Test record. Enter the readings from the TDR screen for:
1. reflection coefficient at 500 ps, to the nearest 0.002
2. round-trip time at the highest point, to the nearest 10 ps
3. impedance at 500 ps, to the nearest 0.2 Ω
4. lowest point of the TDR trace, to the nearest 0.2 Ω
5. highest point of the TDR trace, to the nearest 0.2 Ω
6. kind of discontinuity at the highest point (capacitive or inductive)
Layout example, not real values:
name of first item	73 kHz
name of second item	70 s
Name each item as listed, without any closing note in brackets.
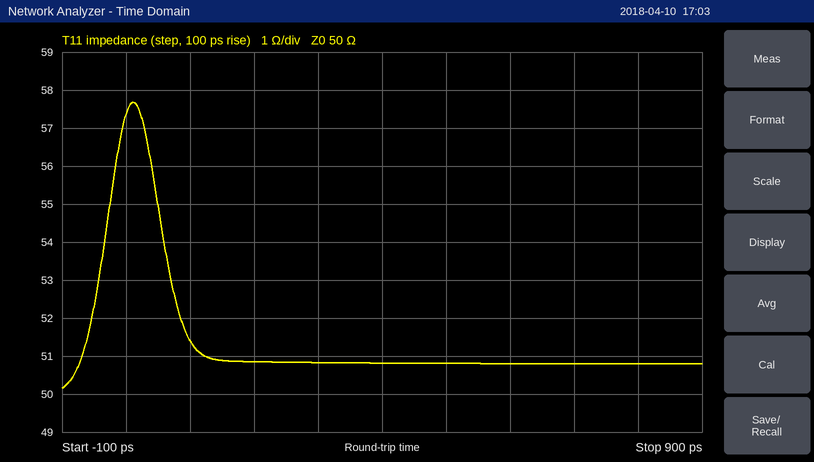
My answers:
reflection coefficient at 500 ps, to the nearest 0.002	+0.008
round-trip time at the highest point, to the nearest 10 ps	10 ps
impedance at 500 ps, to the nearest 0.2 Ω	50.8 Ω
lowest point of the TDR trace, to the nearest 0.2 Ω	50.2 Ω
highest point of the TDR trace, to the nearest 0.2 Ω	57.6 Ω
kind of discontinuity at the highest point	inductive
